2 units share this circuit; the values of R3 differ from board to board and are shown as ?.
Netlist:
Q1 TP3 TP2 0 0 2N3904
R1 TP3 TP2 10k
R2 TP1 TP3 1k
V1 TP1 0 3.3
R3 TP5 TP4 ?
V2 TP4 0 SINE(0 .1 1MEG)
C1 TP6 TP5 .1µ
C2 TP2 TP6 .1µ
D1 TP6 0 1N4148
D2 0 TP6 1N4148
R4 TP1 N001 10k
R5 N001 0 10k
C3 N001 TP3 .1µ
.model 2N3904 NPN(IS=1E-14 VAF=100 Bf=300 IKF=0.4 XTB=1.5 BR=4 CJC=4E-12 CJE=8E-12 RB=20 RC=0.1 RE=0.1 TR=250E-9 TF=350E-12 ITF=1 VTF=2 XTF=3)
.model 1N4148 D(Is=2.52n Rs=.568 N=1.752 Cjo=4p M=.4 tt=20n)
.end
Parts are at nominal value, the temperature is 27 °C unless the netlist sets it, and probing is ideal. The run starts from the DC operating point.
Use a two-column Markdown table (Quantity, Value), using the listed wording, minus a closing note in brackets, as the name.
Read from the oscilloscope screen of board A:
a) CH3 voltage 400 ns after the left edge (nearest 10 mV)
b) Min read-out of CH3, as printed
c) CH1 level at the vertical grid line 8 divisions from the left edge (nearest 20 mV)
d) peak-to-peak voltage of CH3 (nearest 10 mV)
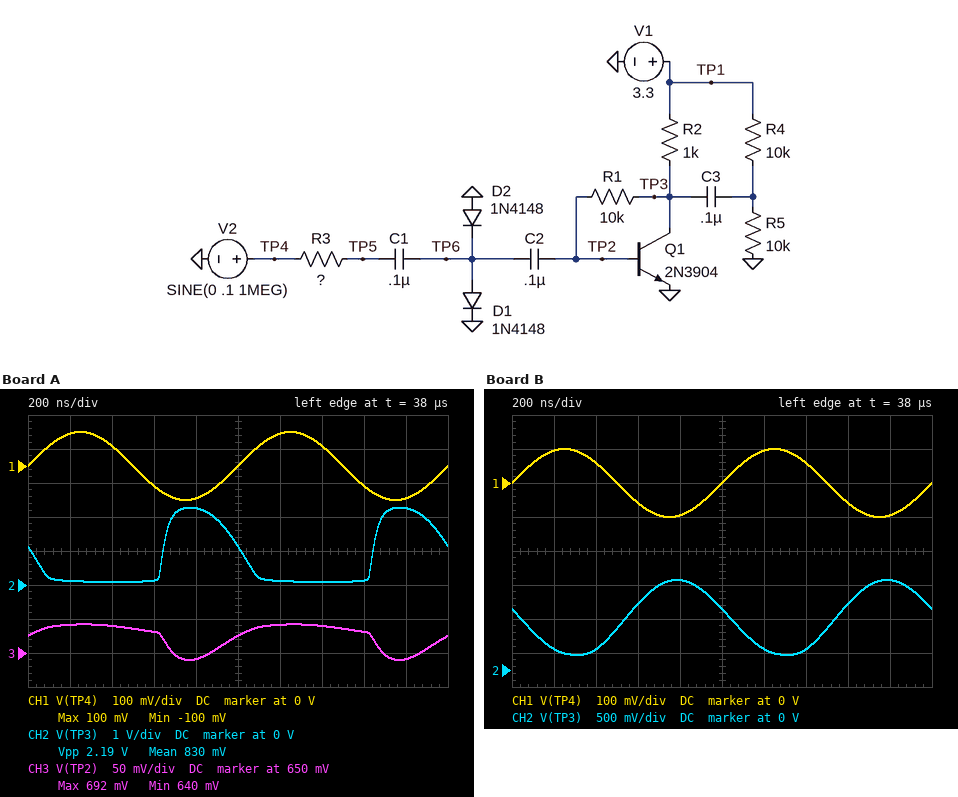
| Quantity | Value |
|---|---|
| CH3 voltage 400 ns after the left edge | 690 mV |
| Min read-out of CH3, as printed | 640 mV |
| CH1 level at the vertical grid line 8 divisions from the left edge | -60 mV |
| peak-to-peak voltage of CH3 | 50 mV |
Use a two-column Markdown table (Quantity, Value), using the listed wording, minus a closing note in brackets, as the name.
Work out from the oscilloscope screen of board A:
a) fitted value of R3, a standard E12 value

| Quantity | Value |
|---|---|
| fitted value of R3, a standard E12 value | 390 Ω |
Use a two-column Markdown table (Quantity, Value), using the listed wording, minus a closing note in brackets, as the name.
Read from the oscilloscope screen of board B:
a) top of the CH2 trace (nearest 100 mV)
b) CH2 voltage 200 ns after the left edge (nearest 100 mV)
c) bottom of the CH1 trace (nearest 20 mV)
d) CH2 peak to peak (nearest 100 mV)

| Quantity | Value |
|---|---|
| top of the CH2 trace | 1.3 V |
| CH2 voltage 200 ns after the left edge | 300 mV |
| bottom of the CH1 trace | -100 mV |
| CH2 peak to peak | 1.1 V |
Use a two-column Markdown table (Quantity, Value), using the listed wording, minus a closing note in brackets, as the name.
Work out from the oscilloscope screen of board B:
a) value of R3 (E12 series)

| Quantity | Value |
|---|---|
| value of R3 | 1.5 kΩ |
